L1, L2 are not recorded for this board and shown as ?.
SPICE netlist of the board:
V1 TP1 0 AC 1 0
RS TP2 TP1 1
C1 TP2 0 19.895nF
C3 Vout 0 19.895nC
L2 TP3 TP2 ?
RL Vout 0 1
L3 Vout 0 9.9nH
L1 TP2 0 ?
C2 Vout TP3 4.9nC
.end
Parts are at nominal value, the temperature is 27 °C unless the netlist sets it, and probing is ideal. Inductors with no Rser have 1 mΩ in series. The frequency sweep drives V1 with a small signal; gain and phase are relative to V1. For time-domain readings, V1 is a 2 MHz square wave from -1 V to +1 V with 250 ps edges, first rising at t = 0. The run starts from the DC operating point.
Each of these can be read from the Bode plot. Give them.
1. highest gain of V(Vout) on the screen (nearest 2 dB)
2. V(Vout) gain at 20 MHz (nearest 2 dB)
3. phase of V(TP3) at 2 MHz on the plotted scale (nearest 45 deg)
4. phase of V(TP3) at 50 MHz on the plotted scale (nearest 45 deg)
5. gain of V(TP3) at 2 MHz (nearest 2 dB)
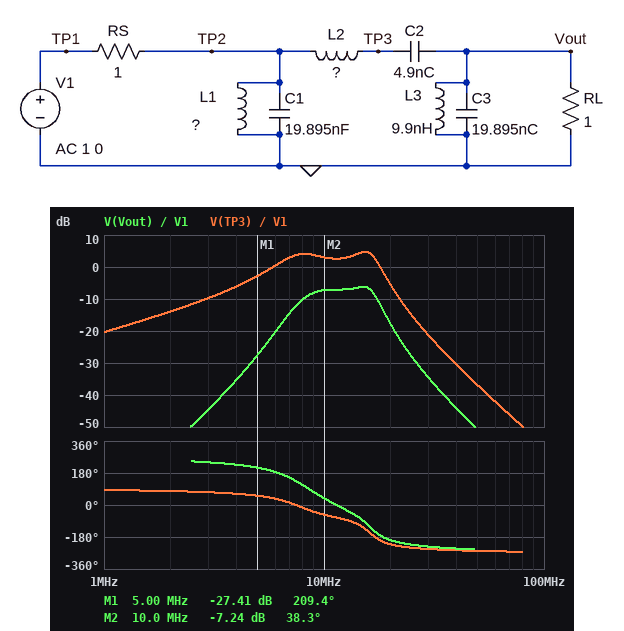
-6 dB
-18 dB
90 deg
-270 deg
-14 dB
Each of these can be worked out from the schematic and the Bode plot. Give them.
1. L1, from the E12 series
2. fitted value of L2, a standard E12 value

15 nH
33 nH
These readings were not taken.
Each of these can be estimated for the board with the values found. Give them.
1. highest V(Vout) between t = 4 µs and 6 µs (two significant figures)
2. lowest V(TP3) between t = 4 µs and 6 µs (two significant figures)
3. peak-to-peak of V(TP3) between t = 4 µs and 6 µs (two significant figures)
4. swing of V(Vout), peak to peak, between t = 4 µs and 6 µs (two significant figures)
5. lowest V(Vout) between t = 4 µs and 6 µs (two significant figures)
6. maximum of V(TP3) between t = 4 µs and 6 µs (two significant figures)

260 mV
-1.4 V
2.9 V
520 mV
-260 mV
1.4 V
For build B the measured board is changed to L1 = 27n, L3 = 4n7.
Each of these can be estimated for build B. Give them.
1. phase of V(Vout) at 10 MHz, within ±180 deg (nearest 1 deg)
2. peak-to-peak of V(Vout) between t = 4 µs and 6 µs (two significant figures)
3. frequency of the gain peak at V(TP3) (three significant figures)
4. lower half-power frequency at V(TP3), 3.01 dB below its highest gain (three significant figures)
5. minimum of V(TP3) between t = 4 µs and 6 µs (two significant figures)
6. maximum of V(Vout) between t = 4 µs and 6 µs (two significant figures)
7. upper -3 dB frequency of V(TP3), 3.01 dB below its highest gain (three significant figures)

86 deg
380 mV
11.7 MHz
5.78 MHz
-1.7 V
190 mV
13.3 MHz
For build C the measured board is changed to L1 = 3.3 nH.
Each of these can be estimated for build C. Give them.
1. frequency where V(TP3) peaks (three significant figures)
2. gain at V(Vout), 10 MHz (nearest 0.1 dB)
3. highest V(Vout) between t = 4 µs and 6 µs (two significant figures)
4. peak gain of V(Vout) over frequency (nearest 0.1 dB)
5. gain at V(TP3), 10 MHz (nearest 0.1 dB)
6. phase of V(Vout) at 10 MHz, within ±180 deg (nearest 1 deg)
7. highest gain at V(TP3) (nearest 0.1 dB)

14.0 MHz
-13.0 dB
170 mV
-8.4 dB
-2.8 dB
126 deg
2.0 dB
